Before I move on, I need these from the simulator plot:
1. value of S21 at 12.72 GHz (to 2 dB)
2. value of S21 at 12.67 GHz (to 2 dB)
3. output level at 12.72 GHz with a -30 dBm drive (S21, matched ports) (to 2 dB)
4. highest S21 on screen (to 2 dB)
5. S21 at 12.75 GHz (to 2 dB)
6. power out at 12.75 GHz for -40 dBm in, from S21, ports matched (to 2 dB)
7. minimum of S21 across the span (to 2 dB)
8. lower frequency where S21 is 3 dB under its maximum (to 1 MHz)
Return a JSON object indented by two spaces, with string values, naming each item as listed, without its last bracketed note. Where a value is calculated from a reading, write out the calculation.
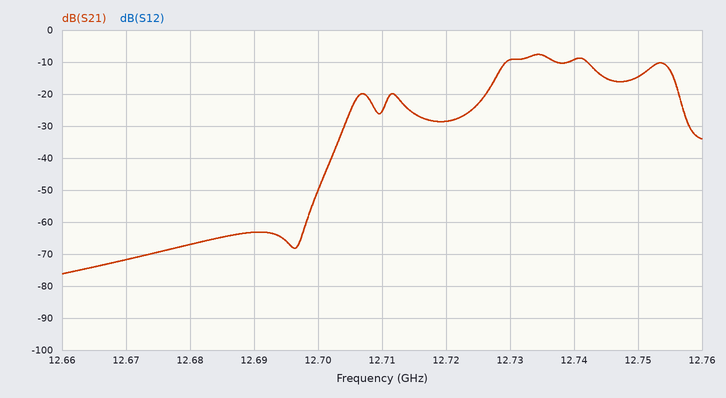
{
  "value of S21 at 12.72 GHz": "-28 dB",
  "value of S21 at 12.67 GHz": "-72 dB",
  "output level at 12.72 GHz with a -30 dBm drive (S21, matched ports)": "-30 dBm + (-28 dB) = -58 dBm",
  "highest S21 on screen": "-8 dB",
  "S21 at 12.75 GHz": "-14 dB",
  "power out at 12.75 GHz for -40 dBm in, from S21, ports matched": "-40 dBm + (-14 dB) = -54 dBm",
  "minimum of S21 across the span": "-76 dB",
  "lower frequency where S21 is 3 dB under its maximum": "12.729 GHz"
}
